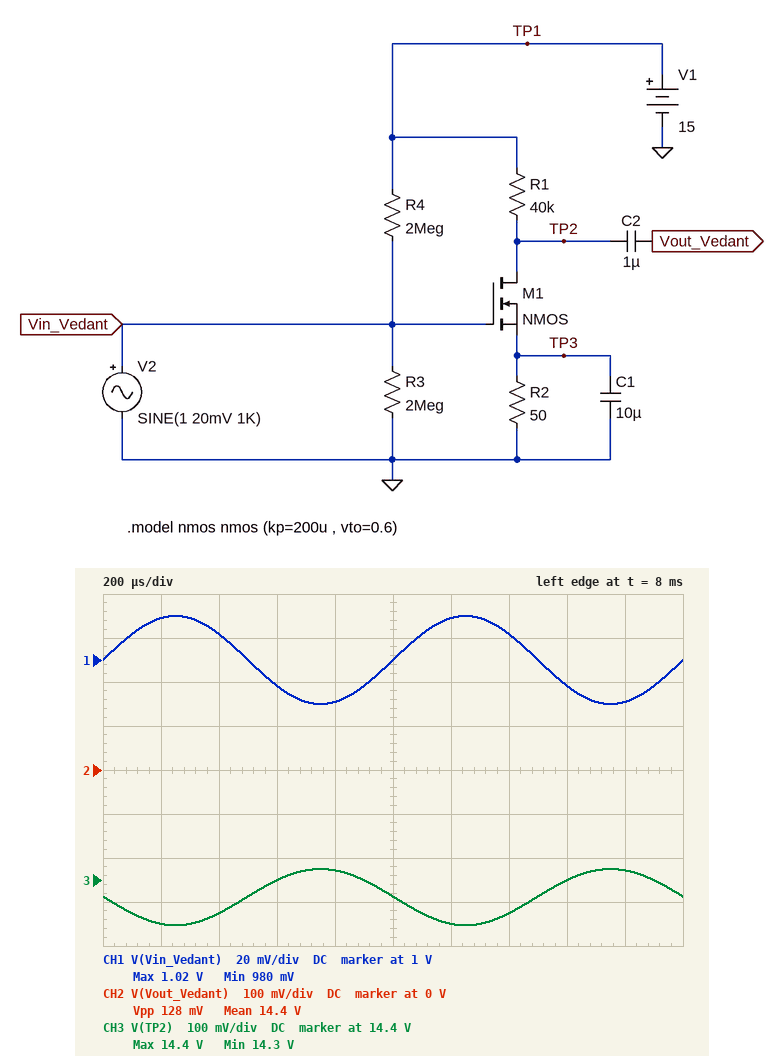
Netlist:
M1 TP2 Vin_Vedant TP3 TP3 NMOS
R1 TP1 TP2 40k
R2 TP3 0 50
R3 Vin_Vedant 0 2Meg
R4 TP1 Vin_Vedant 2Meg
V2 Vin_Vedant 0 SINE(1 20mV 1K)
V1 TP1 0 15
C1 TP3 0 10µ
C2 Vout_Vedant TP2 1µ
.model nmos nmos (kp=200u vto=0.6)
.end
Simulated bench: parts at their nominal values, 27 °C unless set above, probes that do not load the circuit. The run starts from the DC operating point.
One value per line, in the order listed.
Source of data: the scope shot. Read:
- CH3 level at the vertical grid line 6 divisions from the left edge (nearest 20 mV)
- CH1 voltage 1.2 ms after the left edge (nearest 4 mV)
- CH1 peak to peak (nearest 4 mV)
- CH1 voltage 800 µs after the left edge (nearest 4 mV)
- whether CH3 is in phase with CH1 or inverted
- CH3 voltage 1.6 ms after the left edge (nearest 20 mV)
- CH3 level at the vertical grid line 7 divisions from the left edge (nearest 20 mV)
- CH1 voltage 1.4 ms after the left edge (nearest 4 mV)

14.30 V
1.020 V
40 mV
980 mV
inverted
14.40 V
14.32 V
1.012 V
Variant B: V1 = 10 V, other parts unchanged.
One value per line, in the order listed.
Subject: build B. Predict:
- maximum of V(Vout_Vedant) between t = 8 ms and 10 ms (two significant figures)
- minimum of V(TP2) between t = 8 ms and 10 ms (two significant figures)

9.4 V
9.3 V
